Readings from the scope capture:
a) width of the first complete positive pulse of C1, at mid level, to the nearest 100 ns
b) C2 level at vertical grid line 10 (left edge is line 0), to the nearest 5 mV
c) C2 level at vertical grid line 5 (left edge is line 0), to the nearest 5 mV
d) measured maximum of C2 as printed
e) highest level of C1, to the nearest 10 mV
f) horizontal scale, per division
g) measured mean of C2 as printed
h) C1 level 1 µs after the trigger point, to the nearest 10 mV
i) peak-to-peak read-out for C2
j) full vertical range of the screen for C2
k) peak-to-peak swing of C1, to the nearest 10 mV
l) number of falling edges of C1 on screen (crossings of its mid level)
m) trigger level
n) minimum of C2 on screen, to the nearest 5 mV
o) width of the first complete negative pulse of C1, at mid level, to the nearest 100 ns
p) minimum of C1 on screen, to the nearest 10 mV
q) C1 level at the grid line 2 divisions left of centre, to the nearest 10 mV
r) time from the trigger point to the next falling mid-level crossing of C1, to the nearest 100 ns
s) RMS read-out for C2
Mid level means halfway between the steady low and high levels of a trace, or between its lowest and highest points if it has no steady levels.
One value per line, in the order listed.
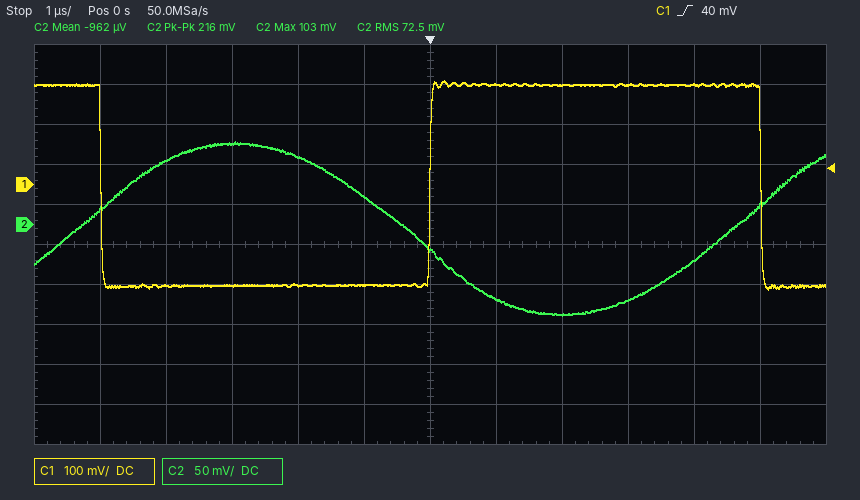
5.0 µs
-45 mV
35 mV
103 mV
260 mV
1 µs
-962 µV
250 mV
216 mV
500 mV
520 mV
2
40 mV
-115 mV
5.0 µs
-260 mV
-250 mV
5.0 µs
72.5 mV
